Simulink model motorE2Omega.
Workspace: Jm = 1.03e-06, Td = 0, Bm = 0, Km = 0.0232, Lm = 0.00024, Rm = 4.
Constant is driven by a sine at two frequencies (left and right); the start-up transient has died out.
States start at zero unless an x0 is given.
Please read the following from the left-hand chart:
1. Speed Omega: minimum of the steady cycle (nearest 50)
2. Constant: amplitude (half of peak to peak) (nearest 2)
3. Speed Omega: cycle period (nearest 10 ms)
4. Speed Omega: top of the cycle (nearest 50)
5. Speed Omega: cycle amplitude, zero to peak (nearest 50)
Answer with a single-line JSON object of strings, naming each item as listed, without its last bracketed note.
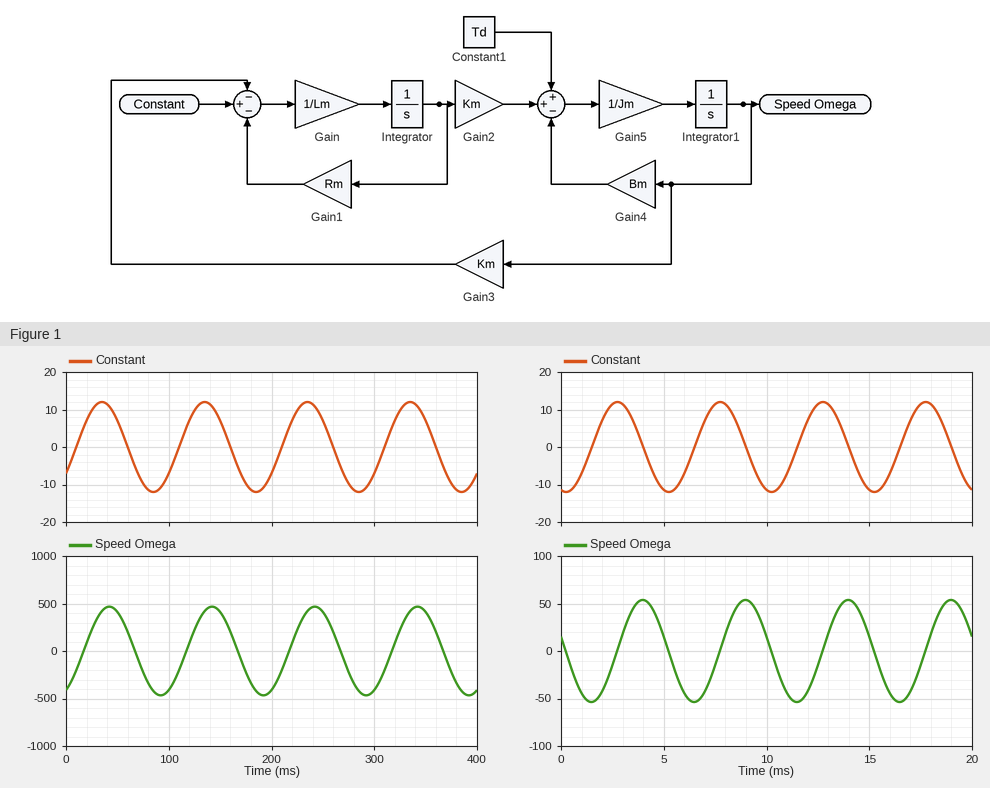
{"Speed Omega: minimum of the steady cycle": "-450", "Constant: amplitude (half of peak to peak)": "12", "Speed Omega: cycle period": "100 ms", "Speed Omega: top of the cycle": "450", "Speed Omega: cycle amplitude, zero to peak": "450"}
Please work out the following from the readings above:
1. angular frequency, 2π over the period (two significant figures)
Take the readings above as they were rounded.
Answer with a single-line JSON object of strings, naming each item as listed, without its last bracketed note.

{"angular frequency, 2π over the period": "0.063 rad/ms"}
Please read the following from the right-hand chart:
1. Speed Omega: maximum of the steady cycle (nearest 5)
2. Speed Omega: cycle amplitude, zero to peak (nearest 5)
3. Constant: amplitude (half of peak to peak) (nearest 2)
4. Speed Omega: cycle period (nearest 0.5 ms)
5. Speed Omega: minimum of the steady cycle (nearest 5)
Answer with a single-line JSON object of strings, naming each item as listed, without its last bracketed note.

{"Speed Omega: maximum of the steady cycle": "55", "Speed Omega: cycle amplitude, zero to peak": "55", "Constant: amplitude (half of peak to peak)": "12", "Speed Omega: cycle period": "5.0 ms", "Speed Omega: minimum of the steady cycle": "-55"}
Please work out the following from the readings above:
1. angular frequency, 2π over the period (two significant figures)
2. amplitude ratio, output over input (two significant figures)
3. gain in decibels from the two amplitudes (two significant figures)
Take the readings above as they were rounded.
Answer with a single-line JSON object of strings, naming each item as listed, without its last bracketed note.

{"angular frequency, 2π over the period": "1.3 rad/ms", "amplitude ratio, output over input": "4.6", "gain in decibels from the two amplitudes": "13 dB"}
